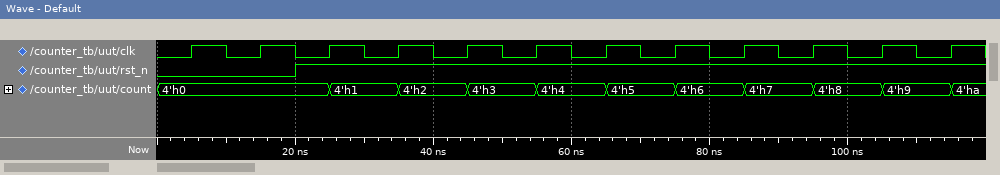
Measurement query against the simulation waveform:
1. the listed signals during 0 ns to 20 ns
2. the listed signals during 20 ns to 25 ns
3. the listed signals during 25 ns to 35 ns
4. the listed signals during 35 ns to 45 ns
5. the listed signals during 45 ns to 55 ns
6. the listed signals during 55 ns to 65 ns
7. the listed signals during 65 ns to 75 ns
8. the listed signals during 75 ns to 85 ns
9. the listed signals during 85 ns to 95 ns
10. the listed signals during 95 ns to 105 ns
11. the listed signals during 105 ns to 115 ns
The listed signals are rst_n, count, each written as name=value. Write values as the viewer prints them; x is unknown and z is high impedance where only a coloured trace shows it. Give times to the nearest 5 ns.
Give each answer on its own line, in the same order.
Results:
rst_n=0, count=4'h0
rst_n=1, count=4'h0
rst_n=1, count=4'h1
rst_n=1, count=4'h2
rst_n=1, count=4'h3
rst_n=1, count=4'h4
rst_n=1, count=4'h5
rst_n=1, count=4'h6
rst_n=1, count=4'h7
rst_n=1, count=4'h8
rst_n=1, count=4'h9
